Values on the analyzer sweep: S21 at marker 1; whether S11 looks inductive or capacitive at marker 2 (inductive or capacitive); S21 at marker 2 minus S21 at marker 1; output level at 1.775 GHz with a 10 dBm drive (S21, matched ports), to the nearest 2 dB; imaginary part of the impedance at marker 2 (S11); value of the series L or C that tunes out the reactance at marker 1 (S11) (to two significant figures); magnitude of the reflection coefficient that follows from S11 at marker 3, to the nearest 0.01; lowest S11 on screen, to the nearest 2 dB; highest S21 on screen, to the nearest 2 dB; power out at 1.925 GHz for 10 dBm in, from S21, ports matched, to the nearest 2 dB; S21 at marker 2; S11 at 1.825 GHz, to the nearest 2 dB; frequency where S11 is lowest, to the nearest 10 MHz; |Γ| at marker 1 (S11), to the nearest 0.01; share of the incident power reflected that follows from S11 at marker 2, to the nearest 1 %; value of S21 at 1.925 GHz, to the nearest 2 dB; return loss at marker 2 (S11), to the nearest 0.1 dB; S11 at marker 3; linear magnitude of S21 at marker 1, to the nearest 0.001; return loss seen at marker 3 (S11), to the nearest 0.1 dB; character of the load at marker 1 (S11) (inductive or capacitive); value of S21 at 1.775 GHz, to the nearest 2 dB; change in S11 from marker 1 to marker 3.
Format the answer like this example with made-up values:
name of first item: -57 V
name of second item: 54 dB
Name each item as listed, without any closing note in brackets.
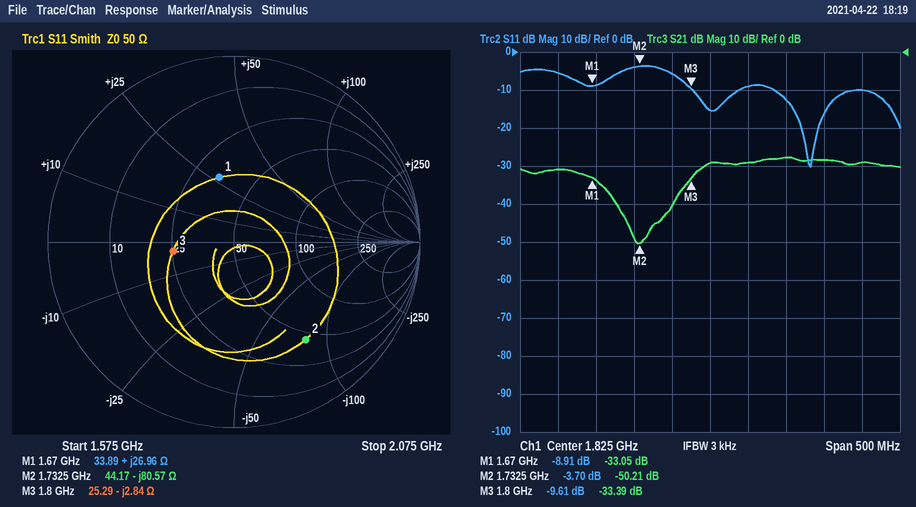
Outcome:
S21 at marker 1: -33.05 dB
whether S11 looks inductive or capacitive at marker 2: capacitive
S21 at marker 2 minus S21 at marker 1: -17.16 dB
output level at 1.775 GHz with a 10 dBm drive (S21, matched ports), to the nearest 2 dB: -30 dBm
imaginary part of the impedance at marker 2: -80.57 Ω
value of the series L or C that tunes out the reactance at marker 1 (S11): 3.5 pF
magnitude of the reflection coefficient that follows from S11 at marker 3, to the nearest 0.01: 0.33
lowest S11 on screen, to the nearest 2 dB: -30 dB
highest S21 on screen, to the nearest 2 dB: -28 dB
power out at 1.925 GHz for 10 dBm in, from S21, ports matched, to the nearest 2 dB: -18 dBm
S21 at marker 2: -50.21 dB
S11 at 1.825 GHz, to the nearest 2 dB: -16 dB
frequency where S11 is lowest, to the nearest 10 MHz: 1.96 GHz
|Γ| at marker 1 (S11), to the nearest 0.01: 0.36
share of the incident power reflected that follows from S11 at marker 2, to the nearest 1 %: 43 %
value of S21 at 1.925 GHz, to the nearest 2 dB: -28 dB
return loss at marker 2 (S11), to the nearest 0.1 dB: 3.7 dB
S11 at marker 3: -9.61 dB
linear magnitude of S21 at marker 1, to the nearest 0.001: 0.022
return loss seen at marker 3 (S11), to the nearest 0.1 dB: 9.6 dB
character of the load at marker 1 (S11): inductive
value of S21 at 1.775 GHz, to the nearest 2 dB: -40 dB
change in S11 from marker 1 to marker 3: -0.70 dB
